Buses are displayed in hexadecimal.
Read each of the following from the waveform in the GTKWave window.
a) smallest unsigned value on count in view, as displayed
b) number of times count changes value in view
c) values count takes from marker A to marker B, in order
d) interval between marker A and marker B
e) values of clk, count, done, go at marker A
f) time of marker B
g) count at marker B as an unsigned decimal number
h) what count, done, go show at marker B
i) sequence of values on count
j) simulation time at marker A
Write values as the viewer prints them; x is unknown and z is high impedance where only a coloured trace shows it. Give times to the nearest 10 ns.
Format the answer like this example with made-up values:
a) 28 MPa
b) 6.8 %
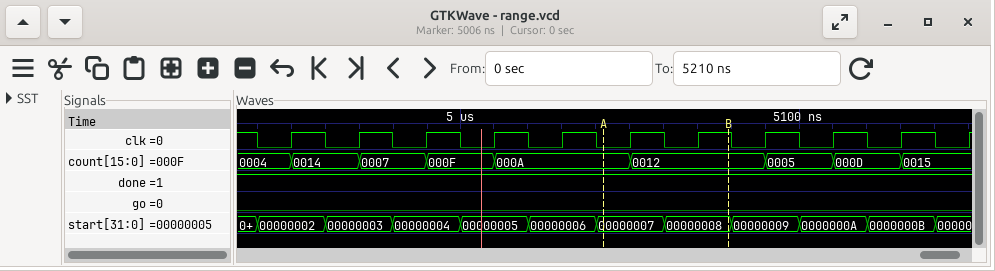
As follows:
a) 0004
b) 8
c) 000A, 0012
d) 40 ns
e) clk=0, count=000A, done=1, go=0
f) 5080 ns
g) 18
h) count=0012, done=1, go=0
i) 0004, 0014, 0007, 000F, 000A, 0012, 0005, 000D, 0015
j) 5040 ns
